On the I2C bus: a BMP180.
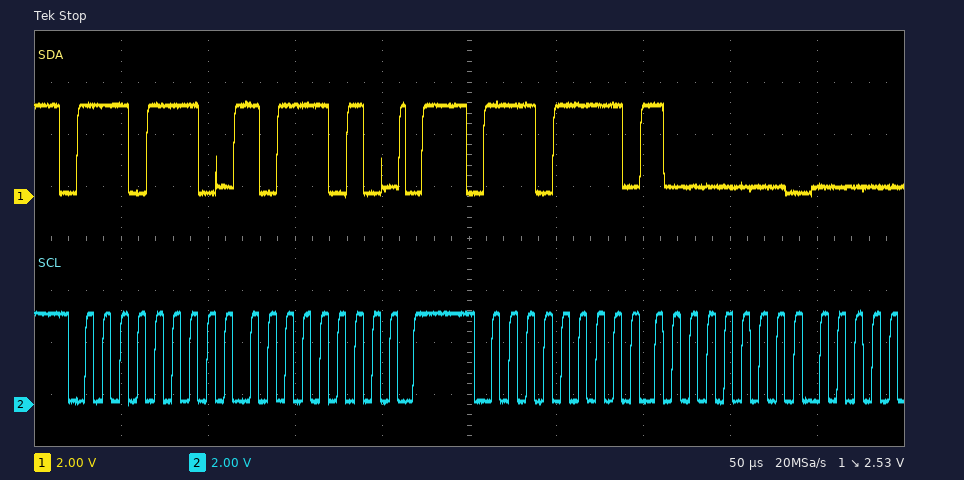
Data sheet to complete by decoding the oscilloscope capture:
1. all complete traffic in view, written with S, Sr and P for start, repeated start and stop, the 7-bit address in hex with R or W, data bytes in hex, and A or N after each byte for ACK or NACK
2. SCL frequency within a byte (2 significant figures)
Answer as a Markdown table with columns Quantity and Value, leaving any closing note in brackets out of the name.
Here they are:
| Quantity | Value |
|---|---|
| all complete traffic in view, written with S, Sr and P for start, repeated start and stop, the 7-bit address in hex with R or W, data bytes in hex, and A or N after each byte for ACK or NACK | S 77W A BA A P S 77R A 80 A |
| SCL frequency within a byte | 100 kHz |
